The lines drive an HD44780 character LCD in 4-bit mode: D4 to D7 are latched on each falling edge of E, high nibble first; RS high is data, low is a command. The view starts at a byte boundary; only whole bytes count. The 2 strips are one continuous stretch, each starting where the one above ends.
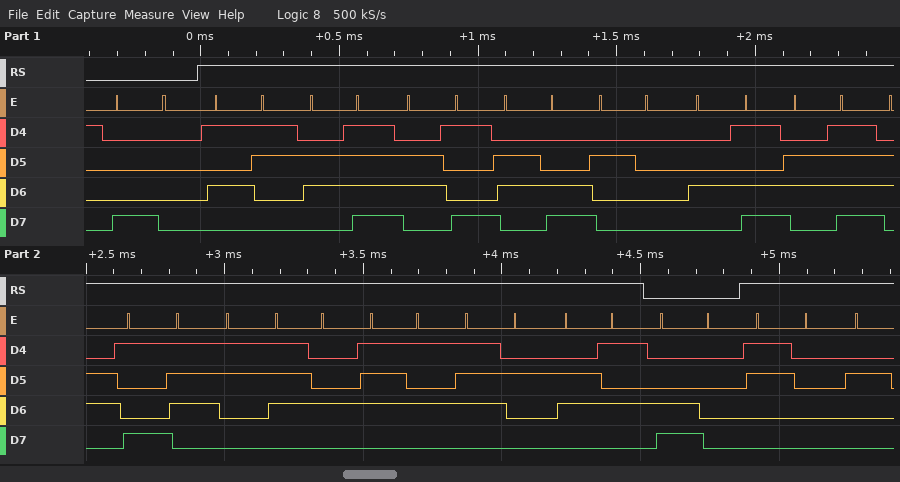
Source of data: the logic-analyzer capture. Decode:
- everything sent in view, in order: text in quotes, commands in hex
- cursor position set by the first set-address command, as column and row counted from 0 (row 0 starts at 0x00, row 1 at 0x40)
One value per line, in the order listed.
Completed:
0x80 "Soil Moisture" 0xC0 "0"
column 0, row 0
